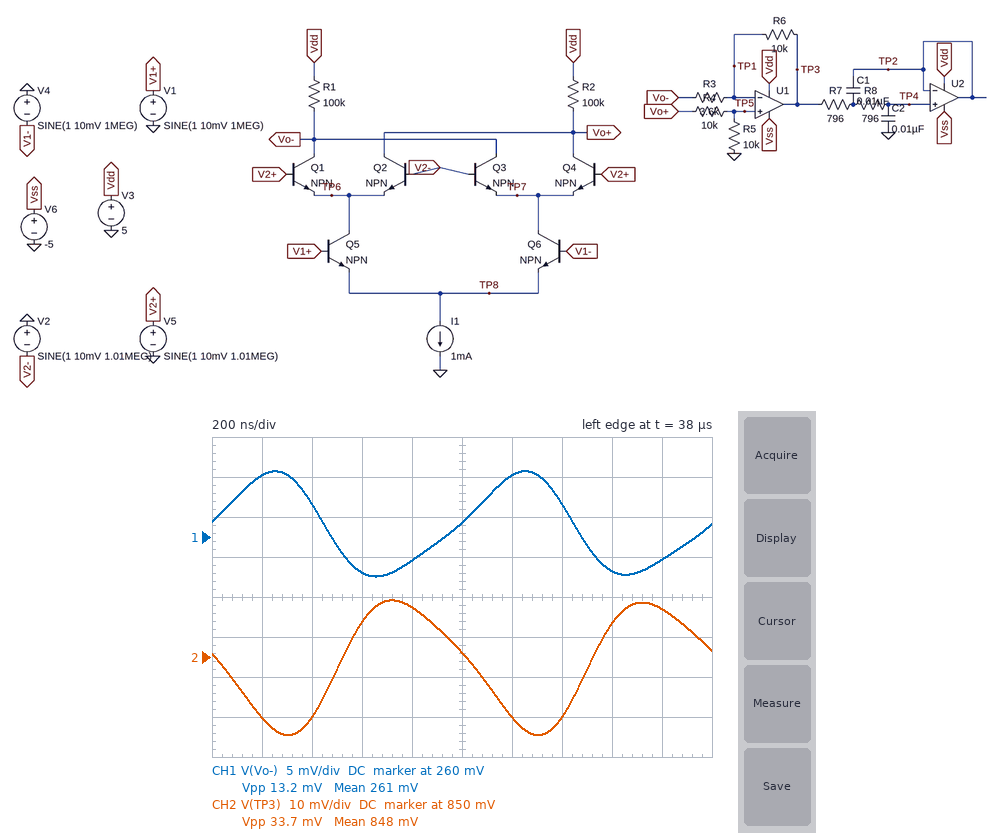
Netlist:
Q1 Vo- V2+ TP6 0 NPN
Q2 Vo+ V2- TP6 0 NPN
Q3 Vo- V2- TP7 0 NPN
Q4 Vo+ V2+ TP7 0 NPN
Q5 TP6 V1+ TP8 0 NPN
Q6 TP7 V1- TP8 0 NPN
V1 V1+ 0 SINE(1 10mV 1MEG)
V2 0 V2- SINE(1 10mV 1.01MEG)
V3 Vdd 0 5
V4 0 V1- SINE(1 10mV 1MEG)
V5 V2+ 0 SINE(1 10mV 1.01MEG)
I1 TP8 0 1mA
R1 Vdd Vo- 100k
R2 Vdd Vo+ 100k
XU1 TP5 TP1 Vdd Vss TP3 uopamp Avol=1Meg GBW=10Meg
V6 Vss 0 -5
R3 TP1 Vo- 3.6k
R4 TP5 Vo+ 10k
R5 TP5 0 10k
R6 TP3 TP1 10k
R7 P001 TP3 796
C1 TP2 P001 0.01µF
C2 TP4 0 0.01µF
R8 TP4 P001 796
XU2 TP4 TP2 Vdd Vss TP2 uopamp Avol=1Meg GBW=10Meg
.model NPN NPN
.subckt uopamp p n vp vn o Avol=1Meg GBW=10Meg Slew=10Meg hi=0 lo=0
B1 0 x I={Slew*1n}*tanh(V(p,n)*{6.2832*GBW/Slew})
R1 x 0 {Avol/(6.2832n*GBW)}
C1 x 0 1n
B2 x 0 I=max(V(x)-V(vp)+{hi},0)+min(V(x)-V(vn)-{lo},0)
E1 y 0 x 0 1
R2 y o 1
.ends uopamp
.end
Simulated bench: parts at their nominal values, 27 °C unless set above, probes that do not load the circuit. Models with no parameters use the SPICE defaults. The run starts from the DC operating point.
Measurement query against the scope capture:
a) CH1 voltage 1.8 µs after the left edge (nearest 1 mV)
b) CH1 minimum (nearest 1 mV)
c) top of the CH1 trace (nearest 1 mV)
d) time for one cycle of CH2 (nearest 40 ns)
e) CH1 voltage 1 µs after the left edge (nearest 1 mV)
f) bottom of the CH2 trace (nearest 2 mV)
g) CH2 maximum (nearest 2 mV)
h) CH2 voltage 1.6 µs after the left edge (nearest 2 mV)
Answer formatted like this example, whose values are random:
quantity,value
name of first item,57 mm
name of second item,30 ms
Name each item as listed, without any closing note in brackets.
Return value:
quantity,value
CH1 voltage 1.8 µs after the left edge,257 mV
CH1 minimum,255 mV
top of the CH1 trace,268 mV
time for one cycle of CH2,1.00 µs
CH1 voltage 1 µs after the left edge,262 mV
bottom of the CH2 trace,830 mV
CH2 maximum,864 mV
CH2 voltage 1.6 µs after the left edge,858 mV
